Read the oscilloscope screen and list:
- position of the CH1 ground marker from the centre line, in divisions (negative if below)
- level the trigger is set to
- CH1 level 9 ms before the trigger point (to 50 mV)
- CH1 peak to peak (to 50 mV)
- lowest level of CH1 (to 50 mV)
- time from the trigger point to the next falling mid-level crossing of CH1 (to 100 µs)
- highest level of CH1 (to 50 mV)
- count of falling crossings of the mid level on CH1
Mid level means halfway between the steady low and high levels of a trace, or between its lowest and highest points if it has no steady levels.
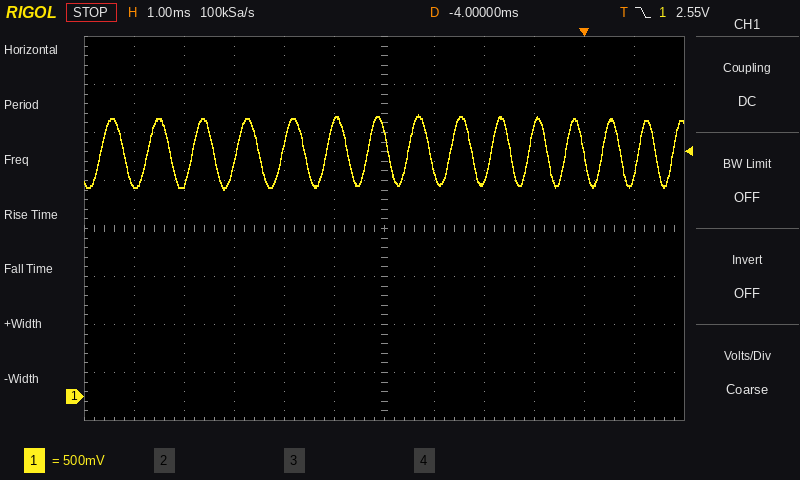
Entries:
-3.5 div
2.55 V
2.20 V
800 mV
2.15 V
700 µs
2.95 V
14
